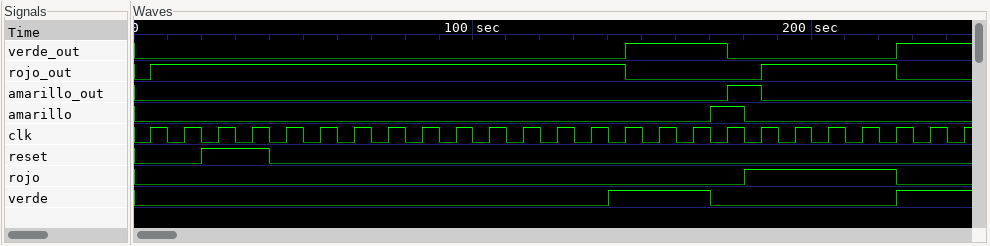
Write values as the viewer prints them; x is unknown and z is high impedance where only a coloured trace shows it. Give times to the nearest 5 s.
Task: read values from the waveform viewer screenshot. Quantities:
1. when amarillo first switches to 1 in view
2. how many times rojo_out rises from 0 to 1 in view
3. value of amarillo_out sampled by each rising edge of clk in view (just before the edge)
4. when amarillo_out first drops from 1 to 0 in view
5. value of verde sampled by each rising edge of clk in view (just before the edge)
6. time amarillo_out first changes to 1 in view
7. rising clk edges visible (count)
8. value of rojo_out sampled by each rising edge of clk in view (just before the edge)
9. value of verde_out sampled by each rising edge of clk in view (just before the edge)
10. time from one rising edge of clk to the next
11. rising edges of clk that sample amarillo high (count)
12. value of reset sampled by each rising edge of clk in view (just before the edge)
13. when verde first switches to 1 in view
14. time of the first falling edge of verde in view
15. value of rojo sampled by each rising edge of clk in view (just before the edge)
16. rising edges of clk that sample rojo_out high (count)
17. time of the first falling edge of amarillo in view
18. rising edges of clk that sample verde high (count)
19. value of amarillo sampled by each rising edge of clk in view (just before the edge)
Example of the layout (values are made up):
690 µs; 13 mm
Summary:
170 s; 2; 0 0 0 0 0 0 0 0 0 0 0 0 0 0 0 0 0 0 1 0 0 0 0 0 0; 185 s; 0 0 0 0 0 0 0 0 0 0 0 0 0 0 1 1 1 0 0 0 0 0 0 1 1; 175 s; 25; 0 1 1 1 1 1 1 1 1 1 1 1 1 1 1 0 0 0 0 1 1 1 1 0 0; 0 0 0 0 0 0 0 0 0 0 0 0 0 0 0 1 1 1 0 0 0 0 0 1 1; 10 s; 1; 0 0 1 1 0 0 0 0 0 0 0 0 0 0 0 0 0 0 0 0 0 0 0 0 0; 140 s; 170 s; 0 0 0 0 0 0 0 0 0 0 0 0 0 0 0 0 0 0 1 1 1 1 1 0 0; 18; 180 s; 5; 0 0 0 0 0 0 0 0 0 0 0 0 0 0 0 0 0 1 0 0 0 0 0 0 0
